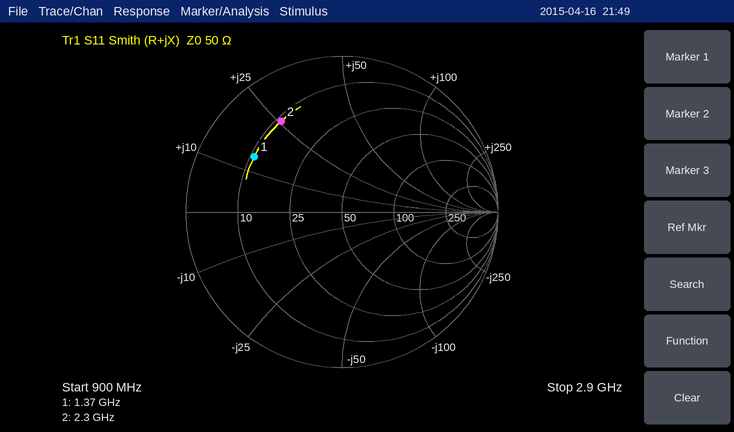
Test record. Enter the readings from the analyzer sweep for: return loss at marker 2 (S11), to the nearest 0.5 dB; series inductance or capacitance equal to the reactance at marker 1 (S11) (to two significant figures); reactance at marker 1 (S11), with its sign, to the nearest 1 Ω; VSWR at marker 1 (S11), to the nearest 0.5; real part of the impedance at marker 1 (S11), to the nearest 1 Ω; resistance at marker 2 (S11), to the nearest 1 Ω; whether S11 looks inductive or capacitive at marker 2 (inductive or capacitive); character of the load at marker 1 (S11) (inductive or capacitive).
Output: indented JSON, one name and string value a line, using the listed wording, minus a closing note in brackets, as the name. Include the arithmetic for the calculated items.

{
  "return loss at marker 2 (S11), to the nearest 0.5 dB": "3.0 dB",
  "series inductance or capacitance equal to the reactance at marker 1 (S11)": "L = 14 Ω/(2π × 1.37 GHz) ≈ 1.6 nH",
  "reactance at marker 1 (S11), with its sign, to the nearest 1 Ω": "+14 Ω",
  "VSWR at marker 1 (S11), to the nearest 0.5": "5.0",
  "real part of the impedance at marker 1 (S11), to the nearest 1 Ω": "11 Ω",
  "resistance at marker 2 (S11), to the nearest 1 Ω": "11 Ω",
  "whether S11 looks inductive or capacitive at marker 2": "inductive",
  "character of the load at marker 1 (S11)": "inductive"
}
